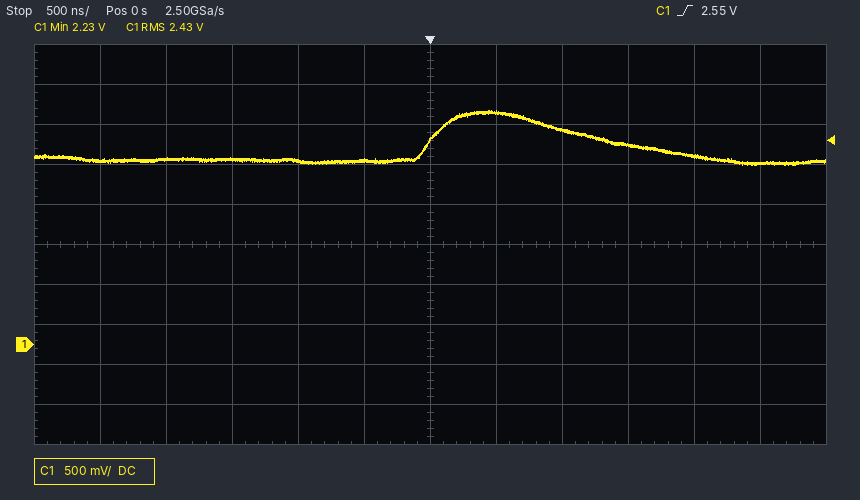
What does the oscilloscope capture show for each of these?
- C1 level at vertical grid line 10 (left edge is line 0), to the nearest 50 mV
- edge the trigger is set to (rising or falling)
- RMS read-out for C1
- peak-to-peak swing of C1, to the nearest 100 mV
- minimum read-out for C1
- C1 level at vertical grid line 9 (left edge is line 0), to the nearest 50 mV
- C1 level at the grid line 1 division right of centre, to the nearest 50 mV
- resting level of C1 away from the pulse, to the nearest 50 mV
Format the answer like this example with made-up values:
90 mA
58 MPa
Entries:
2.35 V
rising
2.43 V
700 mV
2.23 V
2.50 V
2.90 V
2.30 V
